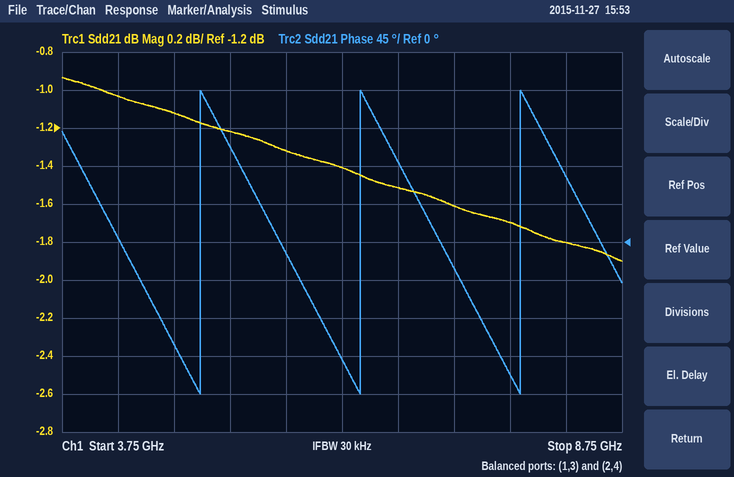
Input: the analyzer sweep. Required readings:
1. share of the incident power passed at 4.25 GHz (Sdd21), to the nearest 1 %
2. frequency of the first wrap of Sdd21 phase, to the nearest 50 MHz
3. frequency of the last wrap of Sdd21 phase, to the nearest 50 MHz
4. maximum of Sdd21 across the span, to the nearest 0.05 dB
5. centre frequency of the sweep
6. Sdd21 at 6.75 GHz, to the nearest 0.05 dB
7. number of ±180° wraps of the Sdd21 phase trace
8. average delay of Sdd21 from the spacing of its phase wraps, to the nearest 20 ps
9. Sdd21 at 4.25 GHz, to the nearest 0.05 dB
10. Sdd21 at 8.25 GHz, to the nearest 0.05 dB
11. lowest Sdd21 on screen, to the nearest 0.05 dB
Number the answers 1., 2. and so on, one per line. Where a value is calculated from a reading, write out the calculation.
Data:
1. 10^(-1.05/10) ≈ 79 %
2. 5.00 GHz
3. 7.85 GHz
4. -0.95 dB
5. 6.25 GHz
6. -1.50 dB
7. 3
8. 2 cycles / (7.85 GHz − 5.00 GHz) ≈ 702 ps, so 700 ps to the nearest 20 ps
9. -1.05 dB
10. -1.80 dB
11. -1.90 dB
